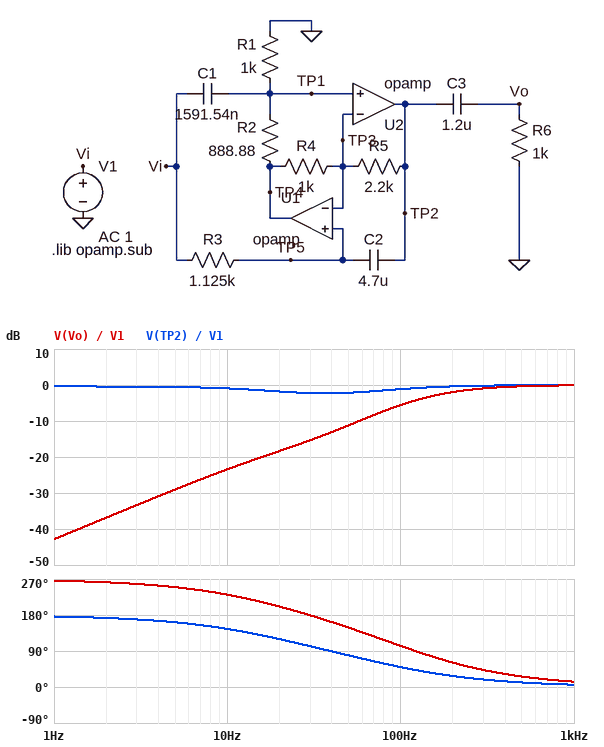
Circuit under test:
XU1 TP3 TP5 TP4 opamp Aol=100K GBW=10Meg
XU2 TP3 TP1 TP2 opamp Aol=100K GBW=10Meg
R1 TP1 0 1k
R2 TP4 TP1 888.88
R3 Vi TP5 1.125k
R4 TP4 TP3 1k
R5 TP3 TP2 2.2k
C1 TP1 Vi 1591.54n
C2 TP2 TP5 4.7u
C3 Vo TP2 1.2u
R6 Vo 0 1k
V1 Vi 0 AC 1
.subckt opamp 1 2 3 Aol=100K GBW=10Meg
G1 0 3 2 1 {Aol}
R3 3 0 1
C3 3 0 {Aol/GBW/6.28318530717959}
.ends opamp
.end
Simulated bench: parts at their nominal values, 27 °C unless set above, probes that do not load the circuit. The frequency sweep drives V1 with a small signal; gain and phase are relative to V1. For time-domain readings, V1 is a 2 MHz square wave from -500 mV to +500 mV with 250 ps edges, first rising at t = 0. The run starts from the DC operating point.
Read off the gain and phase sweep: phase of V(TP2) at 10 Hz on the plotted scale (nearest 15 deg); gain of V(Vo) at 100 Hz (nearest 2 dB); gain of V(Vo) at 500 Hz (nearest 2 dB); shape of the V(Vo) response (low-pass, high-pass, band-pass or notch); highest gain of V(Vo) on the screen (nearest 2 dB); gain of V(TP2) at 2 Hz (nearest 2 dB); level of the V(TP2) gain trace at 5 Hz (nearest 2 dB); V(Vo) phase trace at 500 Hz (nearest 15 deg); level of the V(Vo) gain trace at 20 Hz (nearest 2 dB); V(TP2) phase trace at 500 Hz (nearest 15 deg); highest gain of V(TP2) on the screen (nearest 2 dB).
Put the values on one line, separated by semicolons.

150 deg; -6 dB; 0 dB; high-pass; 0 dB; 0 dB; 0 dB; 30 deg; -18 dB; 15 deg; 0 dB
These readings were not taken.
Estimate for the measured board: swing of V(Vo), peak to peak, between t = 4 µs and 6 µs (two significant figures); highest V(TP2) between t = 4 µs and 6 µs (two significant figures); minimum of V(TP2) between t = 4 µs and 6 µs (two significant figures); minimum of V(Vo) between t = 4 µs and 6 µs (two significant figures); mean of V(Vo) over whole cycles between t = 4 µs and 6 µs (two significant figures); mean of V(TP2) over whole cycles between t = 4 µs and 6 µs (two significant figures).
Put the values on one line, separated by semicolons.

1.5 V; 1.7 V; 230 mV; -250 mV; 500 mV; 980 mV
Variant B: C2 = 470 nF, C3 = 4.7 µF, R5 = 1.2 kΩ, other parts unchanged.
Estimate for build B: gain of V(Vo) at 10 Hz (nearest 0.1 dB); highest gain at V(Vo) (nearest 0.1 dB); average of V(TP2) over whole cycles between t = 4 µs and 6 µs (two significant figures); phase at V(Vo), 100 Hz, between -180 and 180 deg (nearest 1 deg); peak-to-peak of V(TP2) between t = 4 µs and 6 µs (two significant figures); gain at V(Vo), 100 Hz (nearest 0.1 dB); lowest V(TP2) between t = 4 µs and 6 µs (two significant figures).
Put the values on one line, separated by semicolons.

-34.0 dB; 5.2 dB; 530 mV; 170 deg; 1.4 V; -5.3 dB; -190 mV
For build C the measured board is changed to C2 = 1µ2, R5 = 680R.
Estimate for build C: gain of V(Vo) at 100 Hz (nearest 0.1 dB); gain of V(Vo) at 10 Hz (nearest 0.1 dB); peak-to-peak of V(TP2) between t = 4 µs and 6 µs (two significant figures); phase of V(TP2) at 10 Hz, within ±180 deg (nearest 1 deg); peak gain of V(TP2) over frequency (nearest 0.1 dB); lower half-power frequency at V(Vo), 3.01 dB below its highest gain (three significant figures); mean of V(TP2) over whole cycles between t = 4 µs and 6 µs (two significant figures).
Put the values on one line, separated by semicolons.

-20.0 dB; -30.6 dB; 1.4 V; -3 deg; 1.0 dB; 148 Hz; 300 mV
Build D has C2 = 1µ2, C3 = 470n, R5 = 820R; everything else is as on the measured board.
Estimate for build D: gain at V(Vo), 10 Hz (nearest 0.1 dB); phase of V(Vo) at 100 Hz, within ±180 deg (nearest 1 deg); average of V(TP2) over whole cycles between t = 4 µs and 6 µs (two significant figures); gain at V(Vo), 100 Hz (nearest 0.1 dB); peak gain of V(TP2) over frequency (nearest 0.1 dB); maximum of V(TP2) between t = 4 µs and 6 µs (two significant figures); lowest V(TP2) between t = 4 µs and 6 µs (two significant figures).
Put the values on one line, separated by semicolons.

-42.1 dB; -165 deg; 360 mV; -17.4 dB; 1.3 dB; 1.1 V; -330 mV
